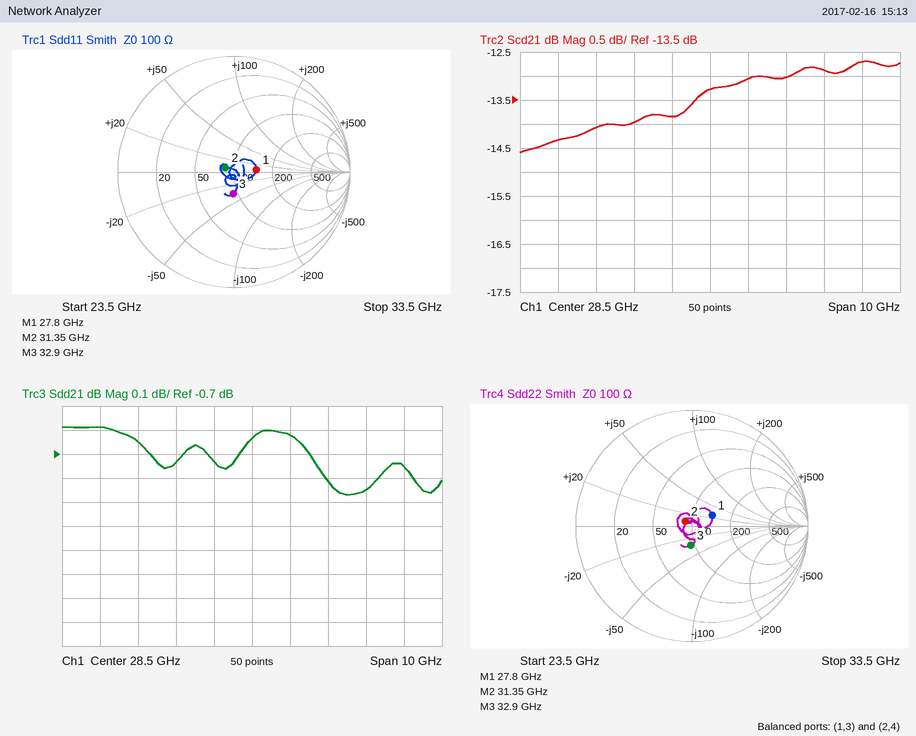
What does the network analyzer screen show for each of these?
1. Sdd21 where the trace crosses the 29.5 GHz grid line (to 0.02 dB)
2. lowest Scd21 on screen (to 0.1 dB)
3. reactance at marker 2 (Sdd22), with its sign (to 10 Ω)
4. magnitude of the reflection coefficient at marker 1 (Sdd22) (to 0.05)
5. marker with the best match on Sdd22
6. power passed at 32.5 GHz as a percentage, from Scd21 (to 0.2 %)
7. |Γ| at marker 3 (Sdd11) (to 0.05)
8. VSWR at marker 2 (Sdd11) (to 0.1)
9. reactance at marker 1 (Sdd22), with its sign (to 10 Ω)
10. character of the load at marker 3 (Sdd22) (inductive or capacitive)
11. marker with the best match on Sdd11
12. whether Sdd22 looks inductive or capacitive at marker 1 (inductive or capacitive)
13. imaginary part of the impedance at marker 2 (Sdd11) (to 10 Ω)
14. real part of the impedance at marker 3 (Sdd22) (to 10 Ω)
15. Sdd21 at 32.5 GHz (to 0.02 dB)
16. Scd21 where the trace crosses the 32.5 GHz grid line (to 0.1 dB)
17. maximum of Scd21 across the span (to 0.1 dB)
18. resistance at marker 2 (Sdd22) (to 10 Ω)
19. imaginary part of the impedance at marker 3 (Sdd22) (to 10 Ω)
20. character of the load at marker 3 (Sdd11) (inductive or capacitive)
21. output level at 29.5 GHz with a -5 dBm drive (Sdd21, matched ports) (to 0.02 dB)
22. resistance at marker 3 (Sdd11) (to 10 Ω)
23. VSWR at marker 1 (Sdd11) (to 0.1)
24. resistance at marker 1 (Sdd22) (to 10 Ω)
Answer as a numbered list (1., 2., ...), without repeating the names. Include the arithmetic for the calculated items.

1. -0.62 dB
2. -14.6 dB
3. +10 Ω
4. 0.20
5. marker 2
6. 10^(-12.7/10) ≈ 5.4 %
7. 0.20
8. 1.2
9. +30 Ω
10. capacitive
11. marker 2
12. inductive
13. +10 Ω
14. 90 Ω
15. -0.76 dB
16. -12.7 dB
17. -12.7 dB
18. 90 Ω
19. -30 Ω
20. capacitive
21. -5 dBm + (-0.62 dB) = -5.62 dBm
22. 90 Ω
23. 1.5
24. 140 Ω
